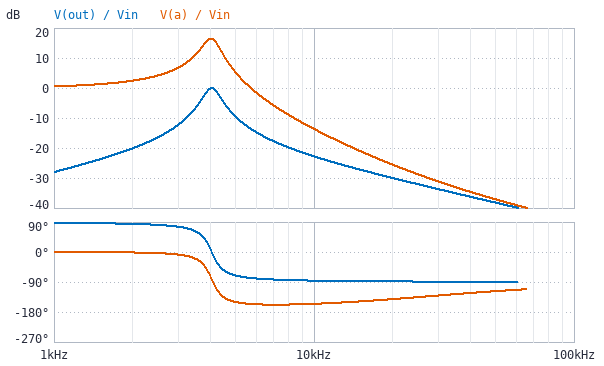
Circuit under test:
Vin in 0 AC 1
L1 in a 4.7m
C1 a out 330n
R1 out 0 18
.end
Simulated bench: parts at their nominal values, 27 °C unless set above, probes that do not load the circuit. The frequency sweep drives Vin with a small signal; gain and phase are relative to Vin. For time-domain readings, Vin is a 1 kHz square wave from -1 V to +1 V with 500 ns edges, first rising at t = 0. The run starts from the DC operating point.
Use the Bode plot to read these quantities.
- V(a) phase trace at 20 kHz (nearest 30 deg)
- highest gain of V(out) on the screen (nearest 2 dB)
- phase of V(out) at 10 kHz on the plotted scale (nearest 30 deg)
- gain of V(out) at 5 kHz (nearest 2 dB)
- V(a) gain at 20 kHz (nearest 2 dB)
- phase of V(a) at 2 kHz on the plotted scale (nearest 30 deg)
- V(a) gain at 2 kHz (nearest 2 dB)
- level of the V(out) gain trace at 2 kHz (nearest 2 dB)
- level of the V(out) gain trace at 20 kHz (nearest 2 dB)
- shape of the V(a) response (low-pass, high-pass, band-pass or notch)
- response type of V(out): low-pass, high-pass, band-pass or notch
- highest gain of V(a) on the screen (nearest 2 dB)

-150 deg
0 dB
-90 deg
-10 dB
-26 dB
0 deg
2 dB
-20 dB
-30 dB
low-pass
band-pass
16 dB
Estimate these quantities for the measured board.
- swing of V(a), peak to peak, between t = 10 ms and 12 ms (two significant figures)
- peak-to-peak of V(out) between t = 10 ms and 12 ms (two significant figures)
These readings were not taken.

4.3 V
390 mV
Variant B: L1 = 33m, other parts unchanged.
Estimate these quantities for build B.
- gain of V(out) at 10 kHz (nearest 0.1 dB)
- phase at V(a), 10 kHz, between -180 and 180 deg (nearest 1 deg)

-41.0 dB
-159 deg
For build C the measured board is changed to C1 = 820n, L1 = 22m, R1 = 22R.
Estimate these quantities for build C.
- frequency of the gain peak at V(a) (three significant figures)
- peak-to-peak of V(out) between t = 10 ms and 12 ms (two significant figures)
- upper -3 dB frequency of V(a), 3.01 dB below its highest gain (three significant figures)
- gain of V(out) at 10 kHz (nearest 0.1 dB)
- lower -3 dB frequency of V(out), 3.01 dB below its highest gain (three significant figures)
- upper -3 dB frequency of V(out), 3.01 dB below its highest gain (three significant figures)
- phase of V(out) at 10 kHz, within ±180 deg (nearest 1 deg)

1.18 kHz
940 mV
1.26 kHz
-35.8 dB
1.11 kHz
1.27 kHz
-89 deg
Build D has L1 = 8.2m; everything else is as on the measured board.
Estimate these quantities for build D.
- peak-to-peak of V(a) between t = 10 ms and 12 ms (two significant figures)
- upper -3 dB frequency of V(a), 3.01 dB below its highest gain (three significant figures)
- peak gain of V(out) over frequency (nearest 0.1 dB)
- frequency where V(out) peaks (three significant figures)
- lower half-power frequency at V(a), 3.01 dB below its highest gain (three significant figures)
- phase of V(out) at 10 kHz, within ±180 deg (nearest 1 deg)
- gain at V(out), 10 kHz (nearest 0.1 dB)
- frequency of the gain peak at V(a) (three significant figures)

9.7 V
3.22 kHz
0 dB
3.06 kHz
2.87 kHz
-88 deg
-28.3 dB
3.05 kHz
